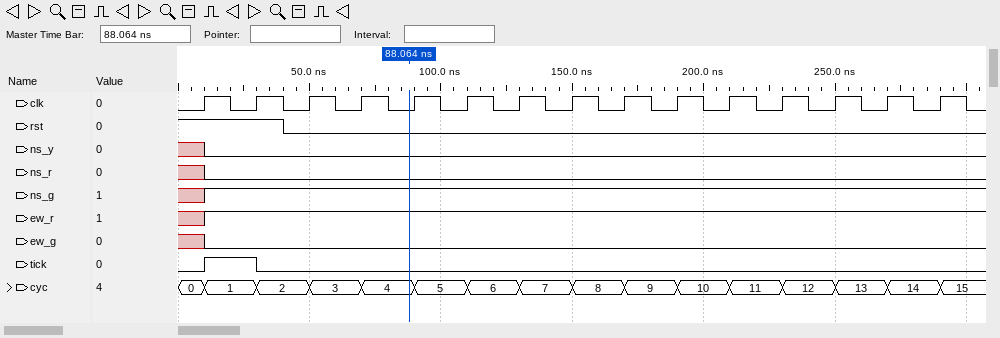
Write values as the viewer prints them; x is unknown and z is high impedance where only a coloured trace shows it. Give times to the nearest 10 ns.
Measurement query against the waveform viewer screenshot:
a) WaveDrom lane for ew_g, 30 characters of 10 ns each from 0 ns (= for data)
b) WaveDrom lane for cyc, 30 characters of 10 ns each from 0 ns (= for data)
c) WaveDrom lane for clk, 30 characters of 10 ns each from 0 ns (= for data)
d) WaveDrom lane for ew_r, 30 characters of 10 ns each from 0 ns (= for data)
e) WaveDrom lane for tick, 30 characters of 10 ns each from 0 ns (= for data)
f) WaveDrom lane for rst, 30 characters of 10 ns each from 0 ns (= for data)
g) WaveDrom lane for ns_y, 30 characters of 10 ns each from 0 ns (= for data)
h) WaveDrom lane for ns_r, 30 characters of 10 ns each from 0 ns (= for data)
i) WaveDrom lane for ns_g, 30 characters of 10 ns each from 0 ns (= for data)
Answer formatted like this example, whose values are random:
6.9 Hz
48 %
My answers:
{name: 'ew_g', wave: 'x0............................'}
{name: 'cyc', wave: '==.=.=.=.=.=.=.=.=.=.=.=.=.=.=', data: '0 1 2 3 4 5 6 7 8 9 10 11 12 13 14 15'}
{name: 'clk', wave: '010101010101010101010101010101'}
{name: 'ew_r', wave: 'x1............................'}
{name: 'tick', wave: '01.0..........................'}
{name: 'rst', wave: '1...0.........................'}
{name: 'ns_y', wave: 'x0............................'}
{name: 'ns_r', wave: 'x0............................'}
{name: 'ns_g', wave: 'x1............................'}
